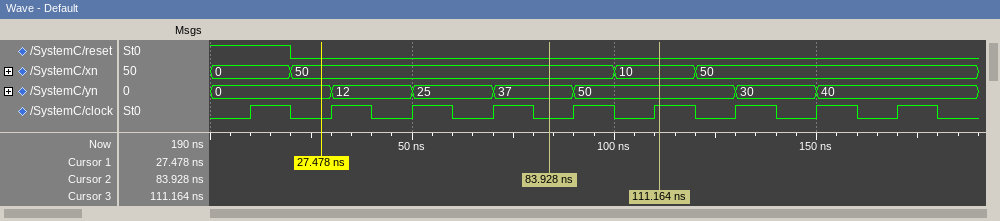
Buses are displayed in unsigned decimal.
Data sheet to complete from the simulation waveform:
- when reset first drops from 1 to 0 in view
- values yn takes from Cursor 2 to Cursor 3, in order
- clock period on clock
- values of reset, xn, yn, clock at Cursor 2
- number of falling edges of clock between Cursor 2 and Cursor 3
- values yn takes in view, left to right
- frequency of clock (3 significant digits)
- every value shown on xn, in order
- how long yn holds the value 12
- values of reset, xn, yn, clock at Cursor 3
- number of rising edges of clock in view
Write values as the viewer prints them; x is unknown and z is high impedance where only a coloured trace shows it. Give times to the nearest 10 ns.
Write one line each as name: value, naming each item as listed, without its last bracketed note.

when reset first drops from 1 to 0 in view: 20 ns
values yn takes from Cursor 2 to Cursor 3, in order: 37, 50
clock period on clock: 20 ns
values of reset, xn, yn, clock at Cursor 2: reset=0, xn=50, yn=37, clock=0
number of falling edges of clock between Cursor 2 and Cursor 3: 1
values yn takes in view, left to right: 0, 12, 25, 37, 50, 30, 40
frequency of clock: 50.0 MHz
every value shown on xn, in order: 0, 50, 10, 50
how long yn holds the value 12: 20 ns
values of reset, xn, yn, clock at Cursor 3: reset=0, xn=10, yn=50, clock=1
number of rising edges of clock in view: 9
